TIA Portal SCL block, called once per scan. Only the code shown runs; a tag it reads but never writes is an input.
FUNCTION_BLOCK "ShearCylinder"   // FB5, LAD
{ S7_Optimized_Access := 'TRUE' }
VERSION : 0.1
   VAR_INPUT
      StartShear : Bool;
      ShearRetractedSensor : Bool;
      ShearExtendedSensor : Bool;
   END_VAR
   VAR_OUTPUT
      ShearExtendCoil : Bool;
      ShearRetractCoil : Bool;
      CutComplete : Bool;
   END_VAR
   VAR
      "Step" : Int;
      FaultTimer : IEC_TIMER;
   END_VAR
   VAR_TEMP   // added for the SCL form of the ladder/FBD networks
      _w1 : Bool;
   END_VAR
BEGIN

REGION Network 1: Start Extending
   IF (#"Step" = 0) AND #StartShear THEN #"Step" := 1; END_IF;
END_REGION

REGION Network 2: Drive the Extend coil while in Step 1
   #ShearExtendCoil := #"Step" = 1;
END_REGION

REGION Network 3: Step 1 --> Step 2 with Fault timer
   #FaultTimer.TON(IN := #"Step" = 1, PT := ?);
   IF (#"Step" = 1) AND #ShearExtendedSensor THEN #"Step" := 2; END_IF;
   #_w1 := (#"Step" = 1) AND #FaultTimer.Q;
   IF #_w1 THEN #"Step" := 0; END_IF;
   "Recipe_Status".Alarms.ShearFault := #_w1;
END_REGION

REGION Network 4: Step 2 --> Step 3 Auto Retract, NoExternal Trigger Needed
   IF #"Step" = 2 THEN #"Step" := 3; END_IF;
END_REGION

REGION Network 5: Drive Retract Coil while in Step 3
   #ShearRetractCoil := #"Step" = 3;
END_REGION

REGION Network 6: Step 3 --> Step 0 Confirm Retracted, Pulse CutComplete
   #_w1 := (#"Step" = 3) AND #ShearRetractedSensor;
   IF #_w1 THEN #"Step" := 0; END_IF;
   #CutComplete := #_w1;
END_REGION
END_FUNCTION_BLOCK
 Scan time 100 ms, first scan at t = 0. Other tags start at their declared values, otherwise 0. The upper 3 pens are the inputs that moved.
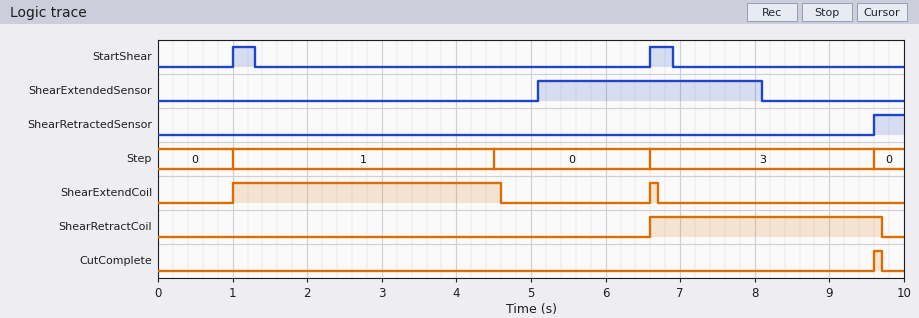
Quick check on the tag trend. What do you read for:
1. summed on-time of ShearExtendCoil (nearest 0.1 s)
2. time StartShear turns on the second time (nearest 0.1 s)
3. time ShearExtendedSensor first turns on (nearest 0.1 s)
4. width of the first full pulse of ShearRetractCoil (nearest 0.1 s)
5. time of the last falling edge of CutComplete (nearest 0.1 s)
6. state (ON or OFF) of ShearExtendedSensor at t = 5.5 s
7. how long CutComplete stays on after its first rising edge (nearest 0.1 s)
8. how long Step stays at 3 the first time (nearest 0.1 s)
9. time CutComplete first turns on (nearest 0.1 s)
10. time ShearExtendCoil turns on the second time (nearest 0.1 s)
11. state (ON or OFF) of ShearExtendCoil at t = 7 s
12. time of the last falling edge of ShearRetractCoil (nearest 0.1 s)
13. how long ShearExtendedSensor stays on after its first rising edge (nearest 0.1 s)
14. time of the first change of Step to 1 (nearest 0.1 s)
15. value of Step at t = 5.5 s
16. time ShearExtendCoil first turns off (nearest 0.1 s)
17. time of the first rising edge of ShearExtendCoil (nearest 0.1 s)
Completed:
3.7 s
6.6 s
5.1 s
3.1 s
9.7 s
ON
0.1 s
3.0 s
9.6 s
6.6 s
OFF
9.7 s
3.0 s
1.0 s
0
4.6 s
1.0 s
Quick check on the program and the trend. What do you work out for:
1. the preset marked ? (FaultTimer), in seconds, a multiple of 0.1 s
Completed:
3.5 s
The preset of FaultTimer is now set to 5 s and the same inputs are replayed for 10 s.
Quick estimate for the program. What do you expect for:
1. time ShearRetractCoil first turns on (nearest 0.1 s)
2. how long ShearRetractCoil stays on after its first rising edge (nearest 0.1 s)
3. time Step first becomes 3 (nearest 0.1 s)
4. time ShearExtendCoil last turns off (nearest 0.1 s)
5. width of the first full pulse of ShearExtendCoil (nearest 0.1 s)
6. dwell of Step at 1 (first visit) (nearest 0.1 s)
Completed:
5.1 s
4.6 s
5.1 s
5.2 s
4.2 s
4.1 s
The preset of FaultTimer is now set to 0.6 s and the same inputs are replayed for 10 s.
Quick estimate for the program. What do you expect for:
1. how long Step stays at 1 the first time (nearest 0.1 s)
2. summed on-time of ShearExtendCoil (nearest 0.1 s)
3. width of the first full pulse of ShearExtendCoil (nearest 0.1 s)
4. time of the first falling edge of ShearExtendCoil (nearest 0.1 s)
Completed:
0.6 s
0.8 s
0.7 s
1.7 s
